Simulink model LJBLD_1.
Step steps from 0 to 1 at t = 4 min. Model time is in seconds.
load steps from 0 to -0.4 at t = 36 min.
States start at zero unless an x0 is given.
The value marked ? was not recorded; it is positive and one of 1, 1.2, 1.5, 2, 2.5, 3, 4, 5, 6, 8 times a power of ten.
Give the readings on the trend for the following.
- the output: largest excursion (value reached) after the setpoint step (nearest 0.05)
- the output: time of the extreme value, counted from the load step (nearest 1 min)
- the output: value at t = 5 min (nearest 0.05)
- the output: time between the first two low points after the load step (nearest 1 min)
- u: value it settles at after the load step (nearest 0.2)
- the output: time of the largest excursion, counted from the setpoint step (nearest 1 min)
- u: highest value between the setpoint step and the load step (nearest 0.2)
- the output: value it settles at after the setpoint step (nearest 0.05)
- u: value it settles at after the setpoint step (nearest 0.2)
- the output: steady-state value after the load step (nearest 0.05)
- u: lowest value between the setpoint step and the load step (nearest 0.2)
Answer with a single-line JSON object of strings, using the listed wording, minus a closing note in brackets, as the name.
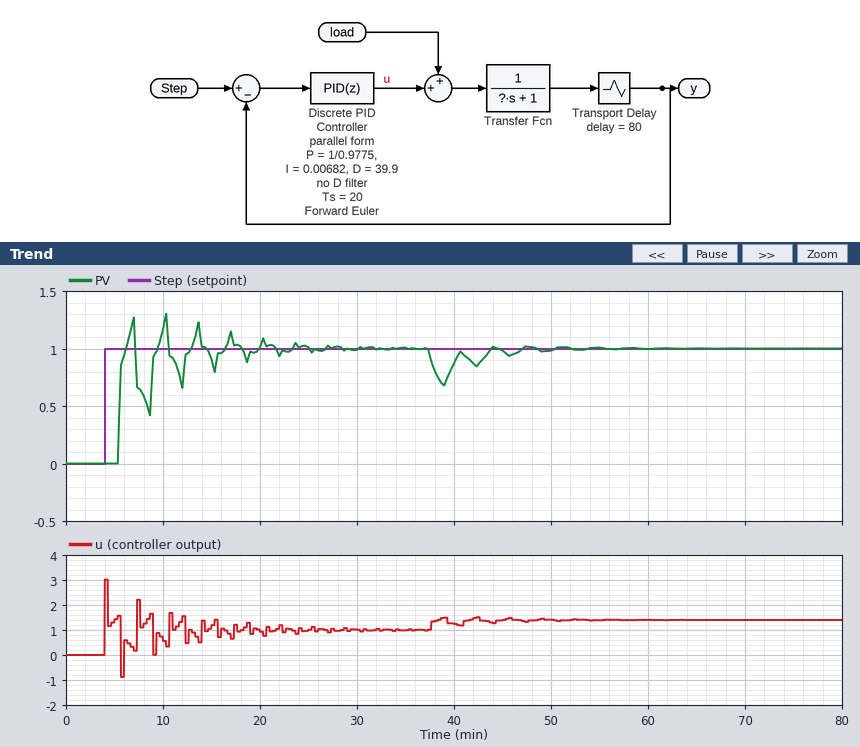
{"the output: largest excursion (value reached) after the setpoint step": "1.30", "the output: time of the extreme value, counted from the load step": "3 min", "the output: value at t = 5 min": "0.00", "the output: time between the first two low points after the load step": "3 min", "u: value it settles at after the load step": "1.4", "the output: time of the largest excursion, counted from the setpoint step": "6 min", "u: highest value between the setpoint step and the load step": "3.0", "the output: value it settles at after the setpoint step": "1.00", "u: value it settles at after the setpoint step": "1.0", "the output: steady-state value after the load step": "1.00", "u: lowest value between the setpoint step and the load step": "-0.8"}
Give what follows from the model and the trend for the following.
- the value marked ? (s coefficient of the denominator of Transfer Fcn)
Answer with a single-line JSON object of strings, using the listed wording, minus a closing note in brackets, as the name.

{"the value marked ?": "60"}
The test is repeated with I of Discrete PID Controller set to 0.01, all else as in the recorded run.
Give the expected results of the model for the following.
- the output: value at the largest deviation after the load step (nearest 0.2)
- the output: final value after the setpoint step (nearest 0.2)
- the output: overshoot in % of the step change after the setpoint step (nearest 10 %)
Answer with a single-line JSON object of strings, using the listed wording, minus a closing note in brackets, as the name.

{"the output: value at the largest deviation after the load step": "0.6", "the output: final value after the setpoint step": "1.0", "the output: overshoot in % of the step change after the setpoint step": "40 %"}
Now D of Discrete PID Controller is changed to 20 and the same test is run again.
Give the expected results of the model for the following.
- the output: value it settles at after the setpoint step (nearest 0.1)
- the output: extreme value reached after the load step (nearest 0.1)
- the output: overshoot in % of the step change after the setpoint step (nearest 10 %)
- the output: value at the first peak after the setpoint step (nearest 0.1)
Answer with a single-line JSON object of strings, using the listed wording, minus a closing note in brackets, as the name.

{"the output: value it settles at after the setpoint step": "1.0", "the output: extreme value reached after the load step": "0.7", "the output: overshoot in % of the step change after the setpoint step": "20 %", "the output: value at the first peak after the setpoint step": "1.2"}
